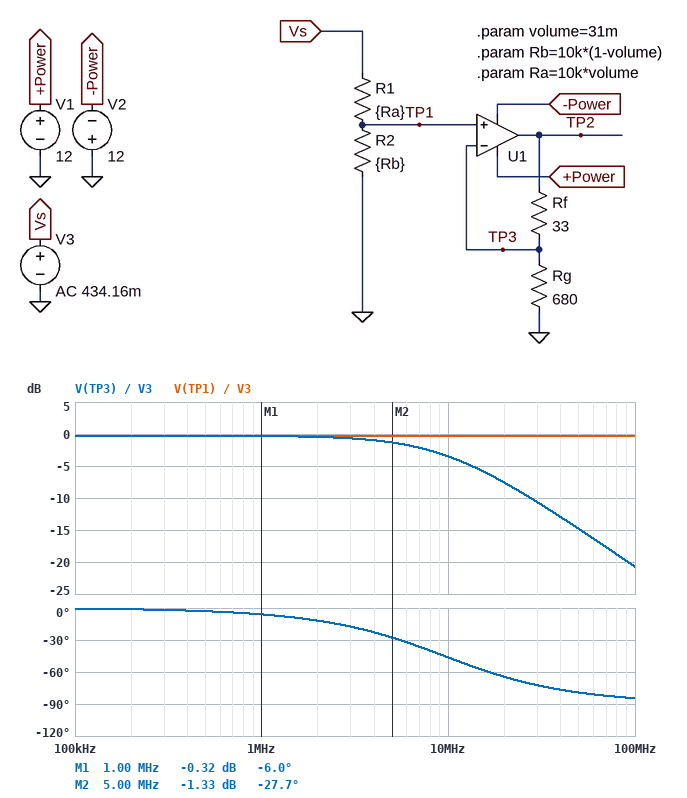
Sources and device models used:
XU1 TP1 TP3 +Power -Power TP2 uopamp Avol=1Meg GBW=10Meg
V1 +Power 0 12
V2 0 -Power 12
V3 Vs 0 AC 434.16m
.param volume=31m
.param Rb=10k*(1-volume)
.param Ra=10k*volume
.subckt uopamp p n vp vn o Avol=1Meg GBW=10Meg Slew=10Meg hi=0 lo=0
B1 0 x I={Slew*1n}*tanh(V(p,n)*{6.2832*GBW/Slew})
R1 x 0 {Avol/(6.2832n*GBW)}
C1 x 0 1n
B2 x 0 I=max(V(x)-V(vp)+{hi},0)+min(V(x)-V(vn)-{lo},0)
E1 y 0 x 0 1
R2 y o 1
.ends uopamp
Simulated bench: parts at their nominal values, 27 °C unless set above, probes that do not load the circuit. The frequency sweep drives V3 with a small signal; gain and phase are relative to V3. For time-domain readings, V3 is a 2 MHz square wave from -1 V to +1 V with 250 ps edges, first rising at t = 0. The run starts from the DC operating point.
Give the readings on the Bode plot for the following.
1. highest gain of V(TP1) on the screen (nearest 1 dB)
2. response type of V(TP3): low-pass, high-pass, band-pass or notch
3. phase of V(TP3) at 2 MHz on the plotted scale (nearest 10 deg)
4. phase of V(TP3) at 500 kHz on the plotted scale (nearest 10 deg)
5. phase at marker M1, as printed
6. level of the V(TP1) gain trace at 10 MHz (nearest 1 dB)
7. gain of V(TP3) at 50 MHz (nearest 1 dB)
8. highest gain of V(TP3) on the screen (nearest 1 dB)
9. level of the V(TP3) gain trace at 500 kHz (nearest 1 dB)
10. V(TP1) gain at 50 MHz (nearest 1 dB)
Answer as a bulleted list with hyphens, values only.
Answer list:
- 0 dB
- low-pass
- -10 deg
- 0 deg
- -6.0 deg
- 0 dB
- -15 dB
- 0 dB
- 0 dB
- 0 dB
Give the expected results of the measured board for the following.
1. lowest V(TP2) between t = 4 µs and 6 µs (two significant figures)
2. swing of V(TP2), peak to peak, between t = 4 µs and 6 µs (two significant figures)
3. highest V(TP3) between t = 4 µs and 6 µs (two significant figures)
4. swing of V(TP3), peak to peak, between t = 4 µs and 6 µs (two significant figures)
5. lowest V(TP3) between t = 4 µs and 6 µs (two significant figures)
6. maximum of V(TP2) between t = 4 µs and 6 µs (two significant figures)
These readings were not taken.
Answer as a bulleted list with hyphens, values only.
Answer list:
- -1.0 V
- 2.0 V
- 960 mV
- 1.9 V
- -960 mV
- 1.0 V
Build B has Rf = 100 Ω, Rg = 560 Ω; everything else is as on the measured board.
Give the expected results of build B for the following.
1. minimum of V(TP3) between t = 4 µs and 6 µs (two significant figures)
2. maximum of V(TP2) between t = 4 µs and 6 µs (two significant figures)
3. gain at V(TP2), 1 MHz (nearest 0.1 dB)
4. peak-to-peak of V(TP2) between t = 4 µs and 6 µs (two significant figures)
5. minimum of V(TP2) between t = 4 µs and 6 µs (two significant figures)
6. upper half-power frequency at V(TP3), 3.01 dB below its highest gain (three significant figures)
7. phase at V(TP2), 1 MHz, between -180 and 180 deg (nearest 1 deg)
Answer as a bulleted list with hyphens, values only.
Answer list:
- -950 mV
- 1.1 V
- 1.1 dB
- 2.2 V
- -1.1 V
- 8.47 MHz
- -7 deg
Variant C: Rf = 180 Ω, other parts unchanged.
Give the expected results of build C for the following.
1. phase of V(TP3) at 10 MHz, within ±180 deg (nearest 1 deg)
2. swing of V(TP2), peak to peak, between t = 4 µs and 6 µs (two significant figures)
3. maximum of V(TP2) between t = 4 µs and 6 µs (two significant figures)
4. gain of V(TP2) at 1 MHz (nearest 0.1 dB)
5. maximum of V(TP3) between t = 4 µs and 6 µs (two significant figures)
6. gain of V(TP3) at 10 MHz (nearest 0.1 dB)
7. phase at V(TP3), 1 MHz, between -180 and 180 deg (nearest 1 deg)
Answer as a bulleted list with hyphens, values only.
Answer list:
- -52 deg
- 2.3 V
- 1.2 V
- 1.7 dB
- 920 mV
- -4.4 dB
- -7 deg
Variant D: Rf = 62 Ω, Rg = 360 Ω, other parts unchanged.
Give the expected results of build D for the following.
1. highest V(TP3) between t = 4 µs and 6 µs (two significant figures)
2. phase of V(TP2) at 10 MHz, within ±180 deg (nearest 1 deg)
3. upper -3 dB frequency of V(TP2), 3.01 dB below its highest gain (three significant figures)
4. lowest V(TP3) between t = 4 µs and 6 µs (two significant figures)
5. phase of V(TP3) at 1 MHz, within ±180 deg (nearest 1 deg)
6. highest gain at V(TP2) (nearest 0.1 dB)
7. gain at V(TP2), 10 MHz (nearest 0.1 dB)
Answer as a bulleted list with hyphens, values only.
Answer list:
- 950 mV
- -50 deg
- 8.51 MHz
- -950 mV
- -7 deg
- 1.1 dB
- -2.7 dB
